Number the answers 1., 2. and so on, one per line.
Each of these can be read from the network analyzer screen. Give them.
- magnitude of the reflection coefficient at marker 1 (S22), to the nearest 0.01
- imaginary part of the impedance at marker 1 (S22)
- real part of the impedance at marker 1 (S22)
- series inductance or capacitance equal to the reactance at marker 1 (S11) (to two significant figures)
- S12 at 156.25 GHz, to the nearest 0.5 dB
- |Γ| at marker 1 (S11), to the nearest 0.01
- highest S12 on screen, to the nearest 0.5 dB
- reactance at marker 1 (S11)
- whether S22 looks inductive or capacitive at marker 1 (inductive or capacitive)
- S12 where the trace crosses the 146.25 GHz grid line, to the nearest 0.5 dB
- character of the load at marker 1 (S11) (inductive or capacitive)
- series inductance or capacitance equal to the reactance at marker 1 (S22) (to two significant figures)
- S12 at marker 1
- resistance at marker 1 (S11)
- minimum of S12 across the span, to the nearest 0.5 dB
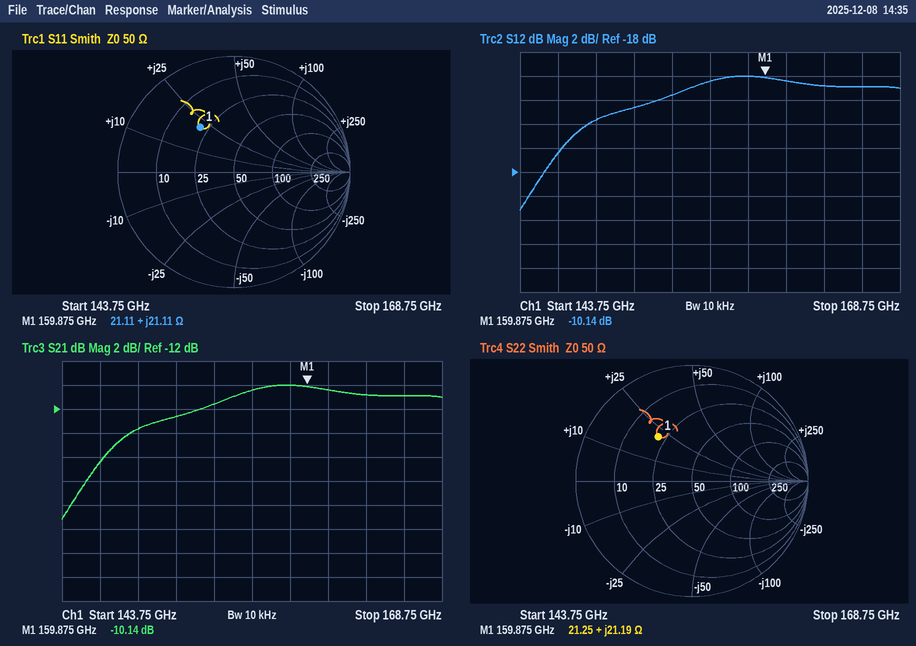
1. 0.48
2. +21.19 Ω
3. 21.25 Ω
4. 21 pH
5. -10.5 dB
6. 0.48
7. -10.0 dB
8. +21.11 Ω
9. inductive
10. -16.5 dB
11. inductive
12. 21 pH
13. -10.14 dB
14. 21.11 Ω
15. -21.0 dB
